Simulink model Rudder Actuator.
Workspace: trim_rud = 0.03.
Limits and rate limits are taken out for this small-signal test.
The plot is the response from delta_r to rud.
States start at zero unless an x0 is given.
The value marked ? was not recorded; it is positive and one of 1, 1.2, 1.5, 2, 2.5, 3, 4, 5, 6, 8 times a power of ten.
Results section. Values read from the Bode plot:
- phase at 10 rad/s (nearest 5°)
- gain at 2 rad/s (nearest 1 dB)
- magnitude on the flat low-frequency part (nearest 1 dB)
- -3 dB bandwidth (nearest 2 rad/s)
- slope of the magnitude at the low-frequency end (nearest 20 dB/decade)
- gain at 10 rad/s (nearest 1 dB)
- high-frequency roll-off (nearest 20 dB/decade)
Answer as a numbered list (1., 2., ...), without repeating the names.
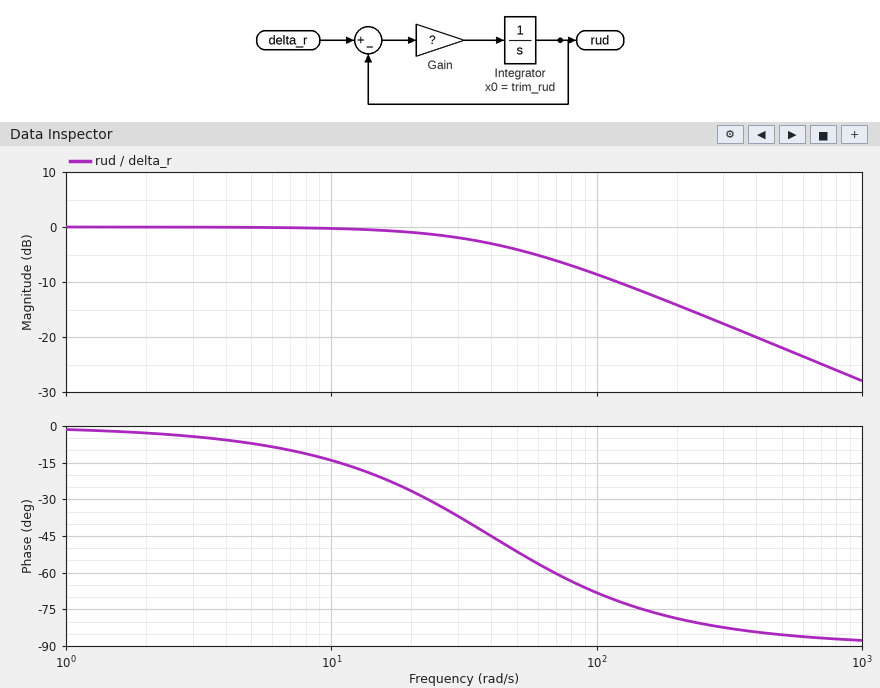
1. -15°
2. 0 dB
3. 0 dB
4. 40 rad/s
5. 0 dB/decade
6. 0 dB
7. -20 dB/decade
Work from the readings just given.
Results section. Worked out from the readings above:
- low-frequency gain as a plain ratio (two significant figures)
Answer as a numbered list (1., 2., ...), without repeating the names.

1. 1.0
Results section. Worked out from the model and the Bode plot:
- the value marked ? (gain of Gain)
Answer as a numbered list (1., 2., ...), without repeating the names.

1. 40
